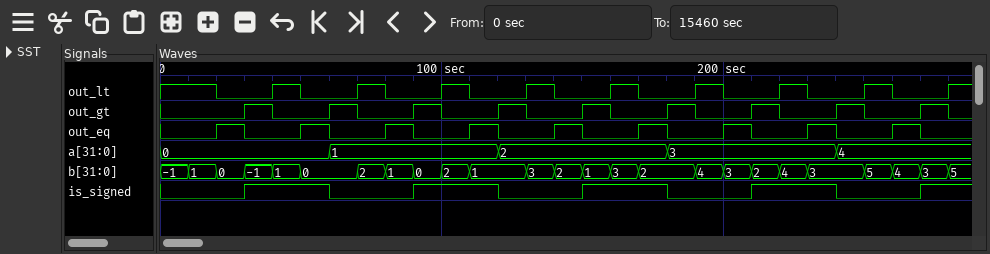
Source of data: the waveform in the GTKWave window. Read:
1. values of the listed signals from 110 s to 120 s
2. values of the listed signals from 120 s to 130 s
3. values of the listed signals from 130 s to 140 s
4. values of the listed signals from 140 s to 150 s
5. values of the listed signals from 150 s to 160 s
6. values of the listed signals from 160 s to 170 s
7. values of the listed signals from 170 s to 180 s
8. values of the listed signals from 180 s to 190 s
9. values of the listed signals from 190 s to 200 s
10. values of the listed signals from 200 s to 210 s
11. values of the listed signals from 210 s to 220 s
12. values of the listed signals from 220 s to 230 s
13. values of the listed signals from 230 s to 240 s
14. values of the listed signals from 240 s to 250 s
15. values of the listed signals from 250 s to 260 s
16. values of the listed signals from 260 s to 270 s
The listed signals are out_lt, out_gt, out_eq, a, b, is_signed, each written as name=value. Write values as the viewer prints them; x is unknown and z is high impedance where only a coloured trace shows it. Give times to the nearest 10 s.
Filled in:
out_lt=0, out_gt=0, out_eq=1, a=1, b=1, is_signed=1
out_lt=0, out_gt=1, out_eq=0, a=2, b=1, is_signed=0
out_lt=1, out_gt=0, out_eq=0, a=2, b=3, is_signed=0
out_lt=0, out_gt=0, out_eq=1, a=2, b=2, is_signed=0
out_lt=0, out_gt=1, out_eq=0, a=2, b=1, is_signed=1
out_lt=1, out_gt=0, out_eq=0, a=2, b=3, is_signed=1
out_lt=0, out_gt=0, out_eq=1, a=2, b=2, is_signed=1
out_lt=0, out_gt=1, out_eq=0, a=3, b=2, is_signed=0
out_lt=1, out_gt=0, out_eq=0, a=3, b=4, is_signed=0
out_lt=0, out_gt=0, out_eq=1, a=3, b=3, is_signed=0
out_lt=0, out_gt=1, out_eq=0, a=3, b=2, is_signed=1
out_lt=1, out_gt=0, out_eq=0, a=3, b=4, is_signed=1
out_lt=0, out_gt=0, out_eq=1, a=3, b=3, is_signed=1
out_lt=0, out_gt=1, out_eq=0, a=4, b=3, is_signed=0
out_lt=1, out_gt=0, out_eq=0, a=4, b=5, is_signed=0
out_lt=0, out_gt=0, out_eq=1, a=4, b=4, is_signed=0
